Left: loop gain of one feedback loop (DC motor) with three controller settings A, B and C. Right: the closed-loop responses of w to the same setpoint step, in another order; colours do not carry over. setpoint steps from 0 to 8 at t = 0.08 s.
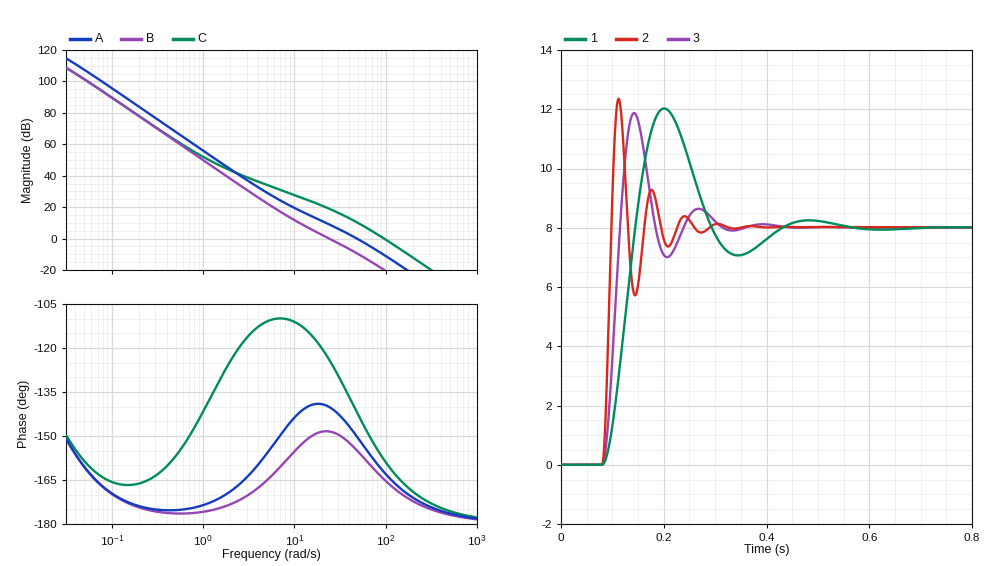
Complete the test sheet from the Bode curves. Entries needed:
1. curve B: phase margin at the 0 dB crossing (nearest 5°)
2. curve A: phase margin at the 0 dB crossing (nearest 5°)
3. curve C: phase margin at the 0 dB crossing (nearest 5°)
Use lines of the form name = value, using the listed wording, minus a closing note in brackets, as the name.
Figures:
curve B: phase margin at the 0 dB crossing = 30°
curve A: phase margin at the 0 dB crossing = 30°
curve C: phase margin at the 0 dB crossing = 20°
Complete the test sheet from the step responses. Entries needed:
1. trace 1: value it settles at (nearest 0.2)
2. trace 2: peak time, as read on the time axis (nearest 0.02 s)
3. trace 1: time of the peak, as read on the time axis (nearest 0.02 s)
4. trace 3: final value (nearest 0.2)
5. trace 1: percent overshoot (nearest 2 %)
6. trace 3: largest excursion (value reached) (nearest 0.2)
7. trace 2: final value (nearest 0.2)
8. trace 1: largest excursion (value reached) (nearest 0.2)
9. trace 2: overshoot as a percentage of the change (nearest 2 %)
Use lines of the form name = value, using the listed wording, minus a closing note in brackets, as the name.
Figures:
trace 1: value it settles at = 8.0
trace 2: peak time, as read on the time axis = 0.12 s
trace 1: time of the peak, as read on the time axis = 0.20 s
trace 3: final value = 8.0
trace 1: percent overshoot = 50 %
trace 3: largest excursion (value reached) = 11.8
trace 2: final value = 8.0
trace 1: largest excursion (value reached) = 12.0
trace 2: overshoot as a percentage of the change = 54 %
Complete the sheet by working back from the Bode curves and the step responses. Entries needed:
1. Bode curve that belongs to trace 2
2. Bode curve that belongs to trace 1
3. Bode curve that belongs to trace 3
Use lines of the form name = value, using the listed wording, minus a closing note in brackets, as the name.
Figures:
Bode curve that belongs to trace 2 = C
Bode curve that belongs to trace 1 = B
Bode curve that belongs to trace 3 = A
